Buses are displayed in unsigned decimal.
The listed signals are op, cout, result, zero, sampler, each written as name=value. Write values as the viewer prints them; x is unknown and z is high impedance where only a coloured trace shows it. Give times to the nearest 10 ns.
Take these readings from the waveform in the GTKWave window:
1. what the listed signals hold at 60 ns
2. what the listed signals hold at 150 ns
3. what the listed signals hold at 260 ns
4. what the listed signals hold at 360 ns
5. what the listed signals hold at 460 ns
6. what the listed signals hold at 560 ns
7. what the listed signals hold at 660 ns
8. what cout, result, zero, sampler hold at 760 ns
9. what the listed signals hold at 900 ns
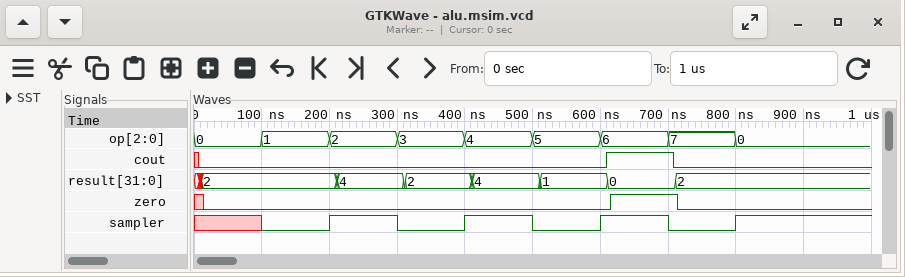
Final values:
op=0, cout=0, result=2, zero=0, sampler=x
op=1, cout=0, result=2, zero=0, sampler=0
op=2, cout=0, result=4, zero=0, sampler=1
op=3, cout=0, result=2, zero=0, sampler=0
op=4, cout=0, result=4, zero=0, sampler=1
op=5, cout=0, result=1, zero=0, sampler=0
op=6, cout=1, result=0, zero=1, sampler=1
cout=0, result=2, zero=0, sampler=0
op=0, cout=0, result=2, zero=0, sampler=1
